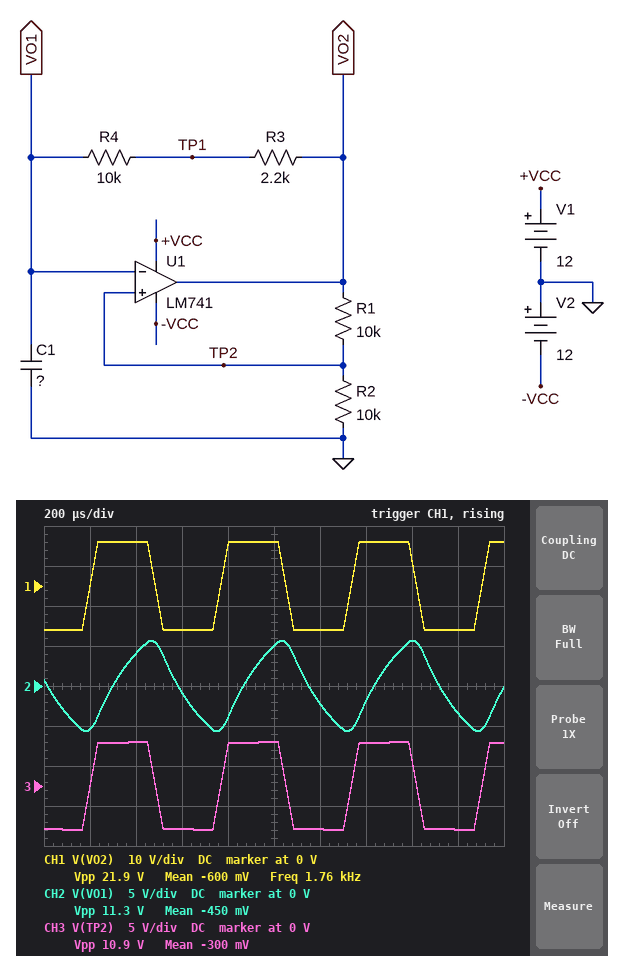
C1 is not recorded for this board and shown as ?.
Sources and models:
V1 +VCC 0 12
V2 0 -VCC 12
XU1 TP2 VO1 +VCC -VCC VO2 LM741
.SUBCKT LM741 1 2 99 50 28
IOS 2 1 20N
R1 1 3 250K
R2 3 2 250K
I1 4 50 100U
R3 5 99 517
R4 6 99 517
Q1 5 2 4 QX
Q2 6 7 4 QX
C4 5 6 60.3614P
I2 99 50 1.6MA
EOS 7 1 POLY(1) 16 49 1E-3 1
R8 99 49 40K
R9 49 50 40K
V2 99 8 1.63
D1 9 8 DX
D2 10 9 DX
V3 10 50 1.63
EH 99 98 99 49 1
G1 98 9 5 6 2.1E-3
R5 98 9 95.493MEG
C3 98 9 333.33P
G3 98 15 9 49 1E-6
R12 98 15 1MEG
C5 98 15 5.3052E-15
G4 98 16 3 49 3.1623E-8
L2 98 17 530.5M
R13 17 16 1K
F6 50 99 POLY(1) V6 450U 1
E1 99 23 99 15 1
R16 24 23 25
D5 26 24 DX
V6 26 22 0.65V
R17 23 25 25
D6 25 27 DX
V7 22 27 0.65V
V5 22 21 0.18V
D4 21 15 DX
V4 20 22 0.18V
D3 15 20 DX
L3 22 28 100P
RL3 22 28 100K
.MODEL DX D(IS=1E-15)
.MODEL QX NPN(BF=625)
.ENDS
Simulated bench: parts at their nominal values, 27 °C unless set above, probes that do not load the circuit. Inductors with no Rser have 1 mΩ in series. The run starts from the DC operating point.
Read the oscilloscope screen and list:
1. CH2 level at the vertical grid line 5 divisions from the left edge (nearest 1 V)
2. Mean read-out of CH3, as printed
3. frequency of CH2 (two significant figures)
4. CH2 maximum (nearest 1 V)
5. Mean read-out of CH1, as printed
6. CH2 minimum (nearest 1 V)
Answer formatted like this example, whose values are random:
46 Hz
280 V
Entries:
5 V
-300 mV
1.8 kHz
6 V
-600 mV
-6 V
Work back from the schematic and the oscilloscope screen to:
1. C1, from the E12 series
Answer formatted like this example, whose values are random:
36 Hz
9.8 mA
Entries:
18 nF
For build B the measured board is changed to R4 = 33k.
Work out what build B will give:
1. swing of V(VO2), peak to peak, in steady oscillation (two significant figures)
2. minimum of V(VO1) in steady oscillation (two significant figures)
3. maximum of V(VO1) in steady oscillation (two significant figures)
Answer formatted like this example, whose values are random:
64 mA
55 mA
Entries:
22 V
-5.5 V
5.5 V
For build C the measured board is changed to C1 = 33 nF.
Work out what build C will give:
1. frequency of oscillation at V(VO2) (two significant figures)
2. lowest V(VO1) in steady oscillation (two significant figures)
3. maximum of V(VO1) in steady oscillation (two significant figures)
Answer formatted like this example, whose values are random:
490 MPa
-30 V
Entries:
1.0 kHz
-5.6 V
5.6 V
